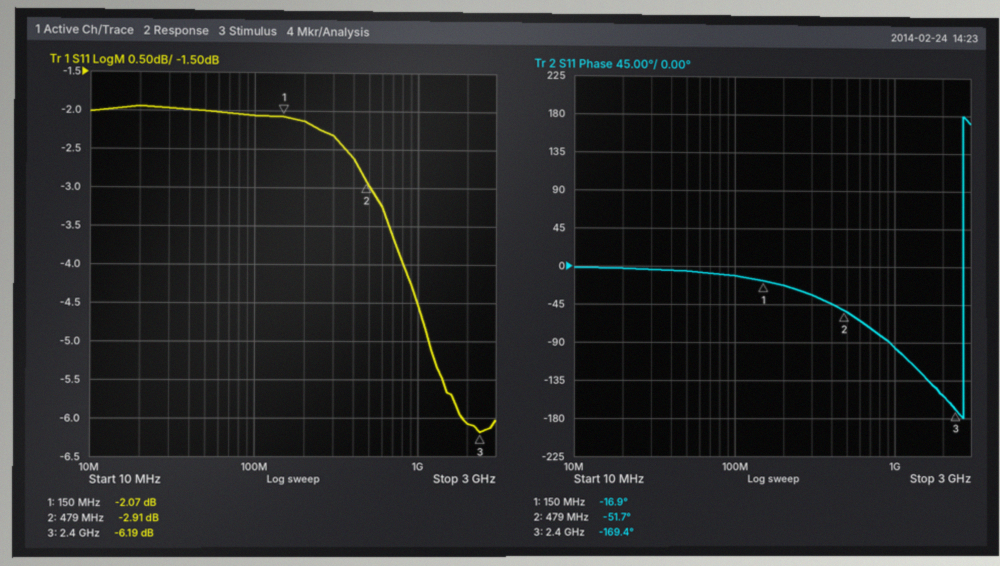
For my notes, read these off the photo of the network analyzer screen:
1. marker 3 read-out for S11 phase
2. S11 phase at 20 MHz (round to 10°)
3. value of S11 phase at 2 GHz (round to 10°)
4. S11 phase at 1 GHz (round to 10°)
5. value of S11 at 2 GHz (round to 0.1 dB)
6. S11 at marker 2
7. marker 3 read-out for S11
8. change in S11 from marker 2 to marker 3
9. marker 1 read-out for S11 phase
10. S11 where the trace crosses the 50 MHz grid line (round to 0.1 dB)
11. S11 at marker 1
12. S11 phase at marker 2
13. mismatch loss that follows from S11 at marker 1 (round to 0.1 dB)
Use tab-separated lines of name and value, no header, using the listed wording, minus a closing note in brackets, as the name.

marker 3 read-out for S11 phase	-169.4°
S11 phase at 20 MHz	0°
value of S11 phase at 2 GHz	-150°
S11 phase at 1 GHz	-100°
value of S11 at 2 GHz	-6.1 dB
S11 at marker 2	-2.91 dB
marker 3 read-out for S11	-6.19 dB
change in S11 from marker 2 to marker 3	-3.28 dB
marker 1 read-out for S11 phase	-16.9°
S11 where the trace crosses the 50 MHz grid line	-2.0 dB
S11 at marker 1	-2.07 dB
S11 phase at marker 2	-51.7°
mismatch loss that follows from S11 at marker 1	4.2 dB
